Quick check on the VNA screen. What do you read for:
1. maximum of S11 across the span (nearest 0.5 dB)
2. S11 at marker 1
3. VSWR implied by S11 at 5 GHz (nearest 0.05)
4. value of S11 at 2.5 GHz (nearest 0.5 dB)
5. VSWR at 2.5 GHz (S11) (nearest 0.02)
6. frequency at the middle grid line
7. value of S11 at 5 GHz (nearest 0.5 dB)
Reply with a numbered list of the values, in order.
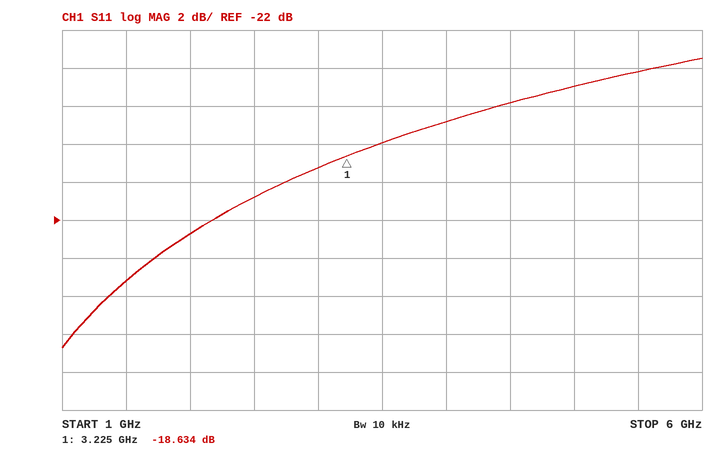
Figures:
1. -13.5 dB
2. -18.634 dB
3. 1.45
4. -21.0 dB
5. 1.20
6. 3.5 GHz
7. -15.0 dB
